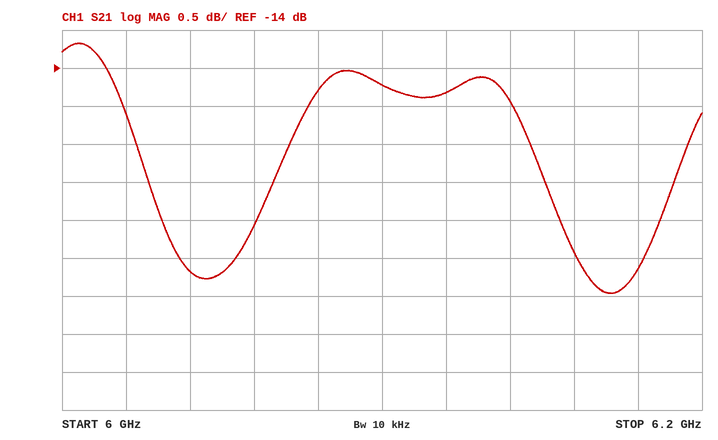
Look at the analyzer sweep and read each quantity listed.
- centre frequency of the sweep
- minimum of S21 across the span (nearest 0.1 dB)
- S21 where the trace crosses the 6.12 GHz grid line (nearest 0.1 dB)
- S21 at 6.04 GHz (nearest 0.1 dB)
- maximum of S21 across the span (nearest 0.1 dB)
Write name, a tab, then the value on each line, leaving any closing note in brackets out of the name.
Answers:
centre frequency of the sweep	6.1 GHz
minimum of S21 across the span	-17.0 dB
S21 where the trace crosses the 6.12 GHz grid line	-14.3 dB
S21 at 6.04 GHz	-16.7 dB
maximum of S21 across the span	-13.7 dB
